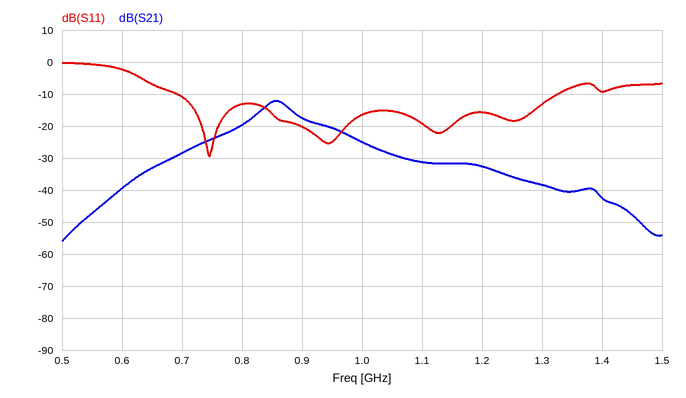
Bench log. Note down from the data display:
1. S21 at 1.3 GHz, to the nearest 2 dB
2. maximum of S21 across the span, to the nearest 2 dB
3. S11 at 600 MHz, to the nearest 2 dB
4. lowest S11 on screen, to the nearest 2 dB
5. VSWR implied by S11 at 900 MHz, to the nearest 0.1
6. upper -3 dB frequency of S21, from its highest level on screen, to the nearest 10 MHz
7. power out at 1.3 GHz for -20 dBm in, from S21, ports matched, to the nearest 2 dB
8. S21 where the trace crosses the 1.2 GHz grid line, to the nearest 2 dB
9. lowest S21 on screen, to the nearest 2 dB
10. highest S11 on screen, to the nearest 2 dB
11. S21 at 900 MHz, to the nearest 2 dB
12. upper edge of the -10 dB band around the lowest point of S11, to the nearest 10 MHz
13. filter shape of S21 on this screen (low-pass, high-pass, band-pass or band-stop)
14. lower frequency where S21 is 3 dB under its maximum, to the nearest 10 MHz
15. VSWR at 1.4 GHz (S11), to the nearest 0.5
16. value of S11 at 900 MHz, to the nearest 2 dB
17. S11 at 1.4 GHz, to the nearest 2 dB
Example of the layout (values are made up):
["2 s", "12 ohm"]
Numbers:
["-38 dB", "-12 dB", "-2 dB", "-30 dB", "1.2", "880 MHz", "-58 dBm", "-32 dB", "-56 dB", "0 dB", "-18 dB", "1.33 GHz", "band-pass", "830 MHz", "2.0", "-20 dB", "-10 dB"]
